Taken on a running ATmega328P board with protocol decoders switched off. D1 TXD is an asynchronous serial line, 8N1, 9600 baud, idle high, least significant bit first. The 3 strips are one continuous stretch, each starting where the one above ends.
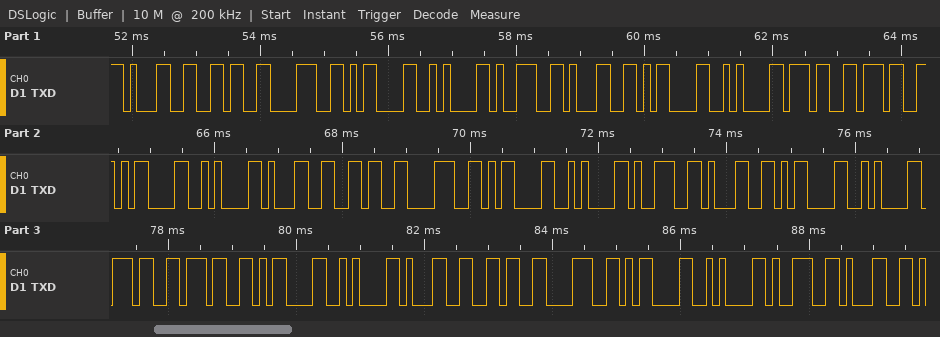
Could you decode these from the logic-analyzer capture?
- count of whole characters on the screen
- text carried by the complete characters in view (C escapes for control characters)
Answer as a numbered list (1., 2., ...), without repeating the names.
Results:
1. 33
2. "168\r\n91\r\n77\r\n168\r\n91\r\n77\r\n168\r\n91"
